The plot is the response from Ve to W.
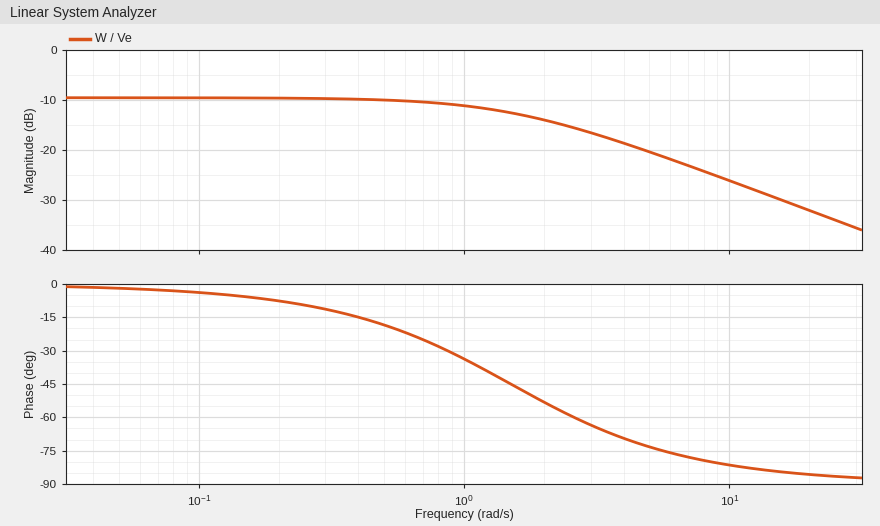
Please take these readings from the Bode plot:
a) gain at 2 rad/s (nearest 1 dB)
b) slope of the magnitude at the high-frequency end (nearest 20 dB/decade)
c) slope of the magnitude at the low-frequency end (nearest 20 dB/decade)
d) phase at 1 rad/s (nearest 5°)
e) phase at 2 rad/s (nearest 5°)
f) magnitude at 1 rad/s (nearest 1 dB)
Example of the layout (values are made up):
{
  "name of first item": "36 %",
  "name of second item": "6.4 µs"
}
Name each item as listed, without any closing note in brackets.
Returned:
{
  "gain at 2 rad/s": "-14 dB",
  "slope of the magnitude at the high-frequency end": "-20 dB/decade",
  "slope of the magnitude at the low-frequency end": "0 dB/decade",
  "phase at 1 rad/s": "-35°",
  "phase at 2 rad/s": "-55°",
  "magnitude at 1 rad/s": "-11 dB"
}
